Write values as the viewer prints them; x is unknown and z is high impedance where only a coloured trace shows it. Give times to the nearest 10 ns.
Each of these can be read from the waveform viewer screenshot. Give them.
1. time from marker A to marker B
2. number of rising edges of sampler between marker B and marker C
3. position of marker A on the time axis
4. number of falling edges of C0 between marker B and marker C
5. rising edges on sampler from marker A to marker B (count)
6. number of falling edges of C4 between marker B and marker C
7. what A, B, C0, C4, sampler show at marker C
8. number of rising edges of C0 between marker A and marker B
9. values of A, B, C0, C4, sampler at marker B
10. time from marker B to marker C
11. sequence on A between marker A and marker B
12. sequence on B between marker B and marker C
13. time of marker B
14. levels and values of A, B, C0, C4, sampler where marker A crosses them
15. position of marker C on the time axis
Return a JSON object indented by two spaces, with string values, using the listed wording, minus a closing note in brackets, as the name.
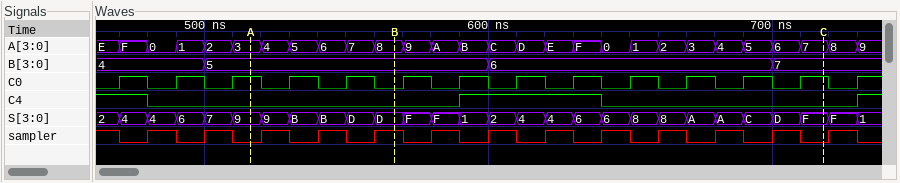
{
  "time from marker A to marker B": "50 ns",
  "number of rising edges of sampler between marker B and marker C": "7",
  "position of marker A on the time axis": "520 ns",
  "number of falling edges of C0 between marker B and marker C": "7",
  "rising edges on sampler from marker A to marker B": "3",
  "number of falling edges of C4 between marker B and marker C": "1",
  "what A, B, C0, C4, sampler show at marker C": "A=7, B=7, C0=1, C4=0, sampler=0",
  "number of rising edges of C0 between marker A and marker B": "2",
  "values of A, B, C0, C4, sampler at marker B": "A=8, B=5, C0=0, C4=0, sampler=1",
  "time from marker B to marker C": "150 ns",
  "sequence on A between marker A and marker B": "3, 4, 5, 6, 7, 8",
  "sequence on B between marker B and marker C": "5, 6, 7",
  "time of marker B": "570 ns",
  "levels and values of A, B, C0, C4, sampler where marker A crosses them": "A=3, B=5, C0=1, C4=0, sampler=0",
  "position of marker C on the time axis": "720 ns"
}
